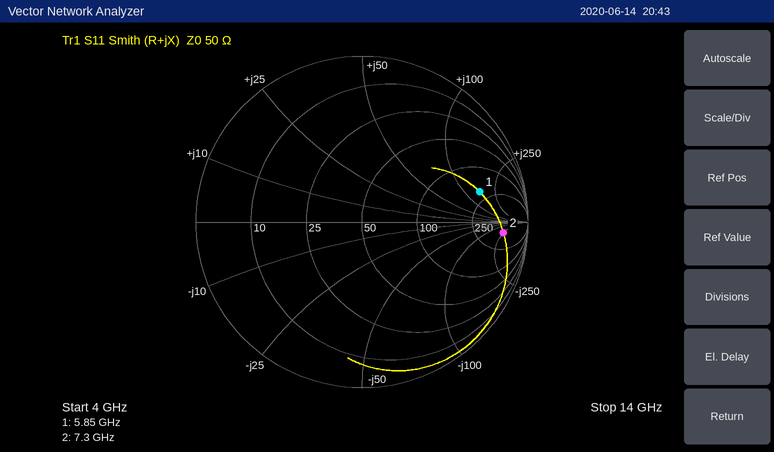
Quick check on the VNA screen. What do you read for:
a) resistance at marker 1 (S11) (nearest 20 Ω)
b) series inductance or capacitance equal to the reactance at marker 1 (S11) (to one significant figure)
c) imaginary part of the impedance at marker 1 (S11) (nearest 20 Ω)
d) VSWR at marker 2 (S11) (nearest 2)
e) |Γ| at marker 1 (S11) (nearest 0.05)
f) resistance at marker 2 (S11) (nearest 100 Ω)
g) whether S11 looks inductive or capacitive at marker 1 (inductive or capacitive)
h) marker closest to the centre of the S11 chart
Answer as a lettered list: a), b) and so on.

a) 200 Ω
b) 4 nH
c) +160 Ω
d) 12
e) 0.75
f) 500 Ω
g) inductive
h) marker 1
